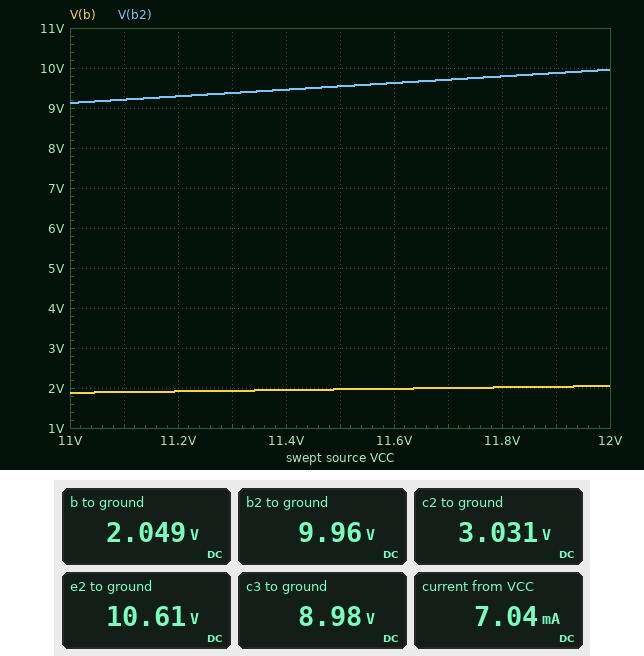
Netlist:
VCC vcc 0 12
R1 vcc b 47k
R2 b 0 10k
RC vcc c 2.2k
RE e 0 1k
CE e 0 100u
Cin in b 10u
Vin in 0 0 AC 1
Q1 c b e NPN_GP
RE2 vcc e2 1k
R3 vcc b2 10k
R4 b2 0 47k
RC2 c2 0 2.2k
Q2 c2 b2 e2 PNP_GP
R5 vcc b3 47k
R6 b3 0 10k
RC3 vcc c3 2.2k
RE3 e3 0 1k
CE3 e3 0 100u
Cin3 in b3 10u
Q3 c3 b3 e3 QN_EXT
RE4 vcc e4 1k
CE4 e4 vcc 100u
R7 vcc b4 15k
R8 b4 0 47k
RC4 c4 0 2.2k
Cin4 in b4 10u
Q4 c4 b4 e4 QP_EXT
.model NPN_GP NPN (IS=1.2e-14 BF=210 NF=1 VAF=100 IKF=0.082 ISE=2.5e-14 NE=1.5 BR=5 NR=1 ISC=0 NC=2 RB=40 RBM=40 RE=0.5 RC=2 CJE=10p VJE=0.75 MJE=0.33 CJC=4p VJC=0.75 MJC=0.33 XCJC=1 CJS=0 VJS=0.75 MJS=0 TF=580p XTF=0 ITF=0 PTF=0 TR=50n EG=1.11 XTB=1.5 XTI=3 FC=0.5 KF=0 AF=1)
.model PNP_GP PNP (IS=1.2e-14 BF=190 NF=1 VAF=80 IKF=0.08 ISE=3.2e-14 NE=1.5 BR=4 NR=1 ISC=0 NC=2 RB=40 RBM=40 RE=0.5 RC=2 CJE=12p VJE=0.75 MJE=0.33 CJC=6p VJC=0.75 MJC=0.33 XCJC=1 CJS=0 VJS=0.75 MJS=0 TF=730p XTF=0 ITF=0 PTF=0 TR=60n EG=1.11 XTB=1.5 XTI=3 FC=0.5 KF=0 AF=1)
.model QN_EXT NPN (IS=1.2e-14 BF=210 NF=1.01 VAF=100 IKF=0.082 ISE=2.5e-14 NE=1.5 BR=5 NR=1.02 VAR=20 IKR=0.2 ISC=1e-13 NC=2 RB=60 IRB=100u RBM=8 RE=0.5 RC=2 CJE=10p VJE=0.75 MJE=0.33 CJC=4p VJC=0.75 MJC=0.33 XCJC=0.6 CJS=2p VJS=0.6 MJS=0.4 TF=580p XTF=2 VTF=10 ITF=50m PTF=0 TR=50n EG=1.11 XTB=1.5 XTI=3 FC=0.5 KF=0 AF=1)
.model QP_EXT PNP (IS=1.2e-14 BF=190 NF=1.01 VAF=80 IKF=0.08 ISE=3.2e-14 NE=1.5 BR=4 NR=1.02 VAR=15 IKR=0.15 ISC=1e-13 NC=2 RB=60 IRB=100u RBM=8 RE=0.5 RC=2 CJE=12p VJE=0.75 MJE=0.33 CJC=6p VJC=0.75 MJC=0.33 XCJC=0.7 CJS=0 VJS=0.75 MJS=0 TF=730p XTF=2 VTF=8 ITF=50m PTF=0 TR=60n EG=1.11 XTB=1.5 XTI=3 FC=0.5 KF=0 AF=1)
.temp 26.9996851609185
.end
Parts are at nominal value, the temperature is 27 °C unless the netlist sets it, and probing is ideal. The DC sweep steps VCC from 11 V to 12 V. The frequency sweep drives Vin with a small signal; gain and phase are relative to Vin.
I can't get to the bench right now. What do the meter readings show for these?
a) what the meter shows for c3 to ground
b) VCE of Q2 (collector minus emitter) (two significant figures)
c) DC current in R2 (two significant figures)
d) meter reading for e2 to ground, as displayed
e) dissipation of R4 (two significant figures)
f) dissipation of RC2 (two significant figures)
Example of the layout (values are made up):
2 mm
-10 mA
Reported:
8.98 V
-7.6 V
200 µA
10.61 V
2.1 mW
4.2 mW
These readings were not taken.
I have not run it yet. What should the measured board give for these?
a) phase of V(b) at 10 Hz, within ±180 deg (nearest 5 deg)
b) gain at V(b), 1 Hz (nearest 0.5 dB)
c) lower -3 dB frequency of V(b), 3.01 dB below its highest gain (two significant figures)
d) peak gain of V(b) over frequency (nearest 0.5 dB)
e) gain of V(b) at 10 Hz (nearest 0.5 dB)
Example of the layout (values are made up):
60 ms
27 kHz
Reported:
10 deg
-7.0 dB
2.1 Hz
0 dB
-0.5 dB
